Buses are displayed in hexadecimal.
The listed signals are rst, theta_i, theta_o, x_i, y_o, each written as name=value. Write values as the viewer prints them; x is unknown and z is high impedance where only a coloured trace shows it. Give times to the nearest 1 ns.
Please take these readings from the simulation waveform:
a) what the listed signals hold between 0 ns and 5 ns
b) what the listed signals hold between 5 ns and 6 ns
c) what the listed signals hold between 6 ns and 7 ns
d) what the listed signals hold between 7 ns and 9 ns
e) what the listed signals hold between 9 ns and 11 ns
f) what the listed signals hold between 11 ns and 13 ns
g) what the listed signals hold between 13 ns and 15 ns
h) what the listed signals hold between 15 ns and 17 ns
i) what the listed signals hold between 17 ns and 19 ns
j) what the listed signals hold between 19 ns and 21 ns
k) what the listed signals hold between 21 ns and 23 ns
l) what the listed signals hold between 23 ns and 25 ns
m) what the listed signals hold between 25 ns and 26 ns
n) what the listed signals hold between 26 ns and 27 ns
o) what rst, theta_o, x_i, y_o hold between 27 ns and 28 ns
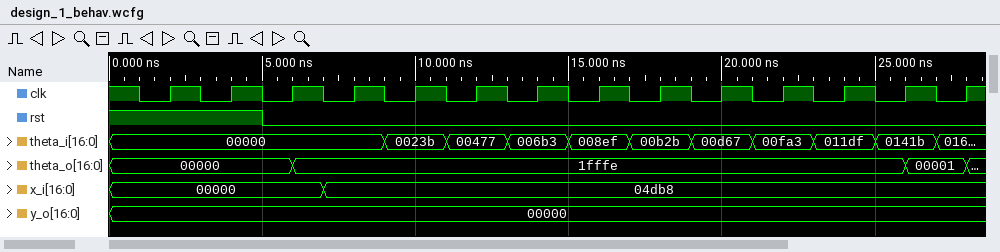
rst=1, theta_i=00000, theta_o=00000, x_i=00000, y_o=00000
rst=0, theta_i=00000, theta_o=00000, x_i=00000, y_o=00000
rst=0, theta_i=00000, theta_o=1fffe, x_i=00000, y_o=00000
rst=0, theta_i=00000, theta_o=1fffe, x_i=04db8, y_o=00000
rst=0, theta_i=0023b, theta_o=1fffe, x_i=04db8, y_o=00000
rst=0, theta_i=00477, theta_o=1fffe, x_i=04db8, y_o=00000
rst=0, theta_i=006b3, theta_o=1fffe, x_i=04db8, y_o=00000
rst=0, theta_i=008ef, theta_o=1fffe, x_i=04db8, y_o=00000
rst=0, theta_i=00b2b, theta_o=1fffe, x_i=04db8, y_o=00000
rst=0, theta_i=00d67, theta_o=1fffe, x_i=04db8, y_o=00000
rst=0, theta_i=00fa3, theta_o=1fffe, x_i=04db8, y_o=00000
rst=0, theta_i=011df, theta_o=1fffe, x_i=04db8, y_o=00000
rst=0, theta_i=0141b, theta_o=1fffe, x_i=04db8, y_o=00000
rst=0, theta_i=0141b, theta_o=00001, x_i=04db8, y_o=00000
rst=0, theta_o=00001, x_i=04db8, y_o=00000
